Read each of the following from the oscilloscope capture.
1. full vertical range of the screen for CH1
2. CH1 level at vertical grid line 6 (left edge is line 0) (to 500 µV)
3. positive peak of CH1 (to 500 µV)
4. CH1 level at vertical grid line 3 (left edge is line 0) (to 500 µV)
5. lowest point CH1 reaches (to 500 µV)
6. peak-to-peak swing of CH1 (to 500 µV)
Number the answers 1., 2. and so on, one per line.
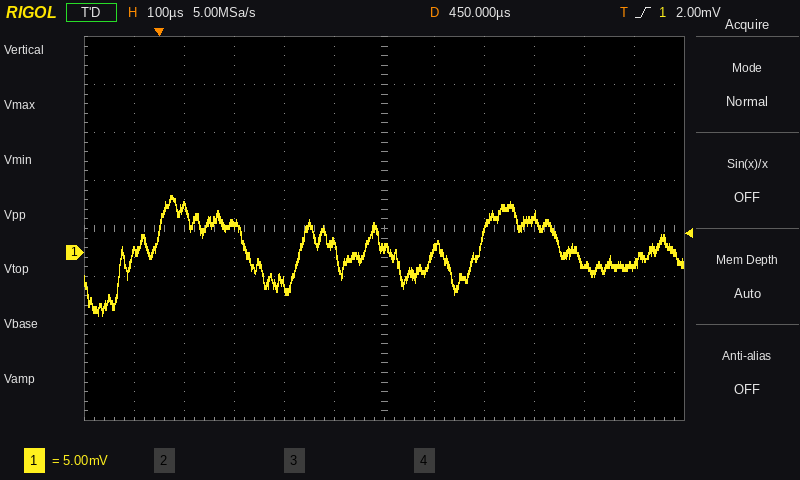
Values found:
1. 40 mV
2. 500 µV
3. 6.0 mV
4. 3.0 mV
5. -6.5 mV
6. 12.5 mV
